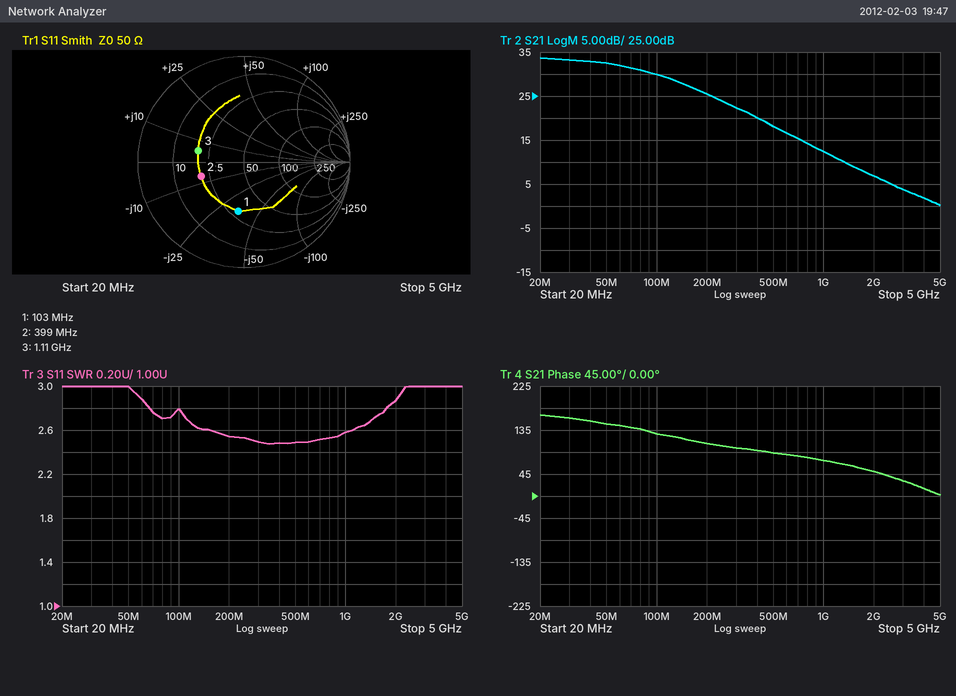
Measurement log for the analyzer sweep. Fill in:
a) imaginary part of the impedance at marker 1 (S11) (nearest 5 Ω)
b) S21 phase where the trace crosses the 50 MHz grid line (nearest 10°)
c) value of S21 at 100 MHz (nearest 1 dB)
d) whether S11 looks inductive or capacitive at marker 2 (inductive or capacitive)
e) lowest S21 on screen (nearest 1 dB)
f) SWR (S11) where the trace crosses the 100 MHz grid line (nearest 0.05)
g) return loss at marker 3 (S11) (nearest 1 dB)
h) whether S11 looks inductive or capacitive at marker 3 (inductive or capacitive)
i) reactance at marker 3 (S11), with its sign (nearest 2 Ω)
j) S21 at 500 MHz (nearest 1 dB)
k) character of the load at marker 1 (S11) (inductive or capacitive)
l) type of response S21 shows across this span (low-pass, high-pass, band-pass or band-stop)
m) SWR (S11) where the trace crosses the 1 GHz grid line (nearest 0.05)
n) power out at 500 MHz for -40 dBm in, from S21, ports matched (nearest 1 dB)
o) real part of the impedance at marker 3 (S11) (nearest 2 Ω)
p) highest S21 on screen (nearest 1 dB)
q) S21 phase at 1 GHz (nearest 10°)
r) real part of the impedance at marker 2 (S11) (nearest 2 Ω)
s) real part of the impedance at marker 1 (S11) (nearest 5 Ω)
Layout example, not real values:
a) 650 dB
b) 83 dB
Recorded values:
a) -35 Ω
b) 150°
c) 30 dB
d) capacitive
e) 0 dB
f) 2.80
g) 7 dB
h) inductive
i) +6 Ω
j) 18 dB
k) capacitive
l) low-pass
m) 2.60
n) -22 dBm
o) 20 Ω
p) 34 dB
q) 70°
r) 20 Ω
s) 30 Ω
